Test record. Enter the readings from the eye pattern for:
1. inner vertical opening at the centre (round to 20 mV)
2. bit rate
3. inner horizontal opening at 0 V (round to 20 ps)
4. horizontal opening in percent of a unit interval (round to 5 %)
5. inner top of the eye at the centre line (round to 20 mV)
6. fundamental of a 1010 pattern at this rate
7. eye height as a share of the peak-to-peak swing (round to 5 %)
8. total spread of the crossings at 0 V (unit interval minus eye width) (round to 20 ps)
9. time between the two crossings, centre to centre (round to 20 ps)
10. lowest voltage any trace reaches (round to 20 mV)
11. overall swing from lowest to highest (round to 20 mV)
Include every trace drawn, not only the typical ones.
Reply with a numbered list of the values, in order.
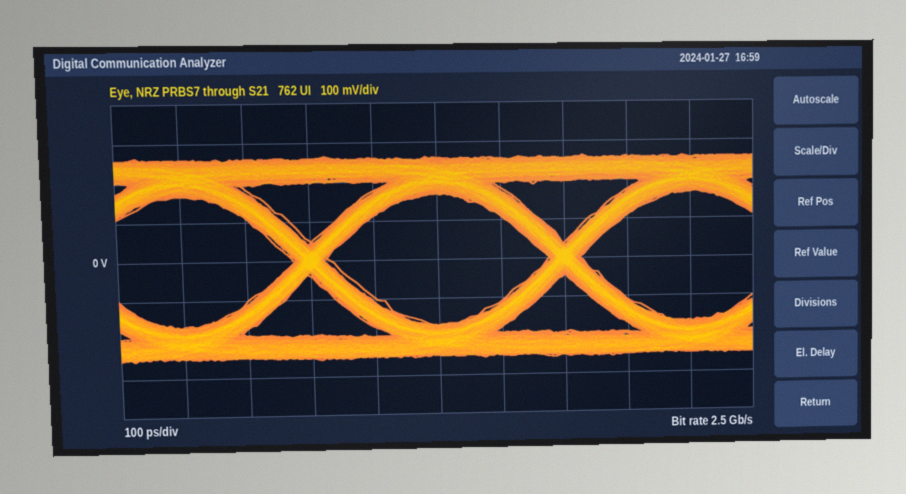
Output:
1. 340 mV
2. 2.5 Gb/s
3. 340 ps
4. 85 %
5. 160 mV
6. 1.25 GHz
7. 65 %
8. 60 ps
9. 400 ps
10. -260 mV
11. 520 mV
